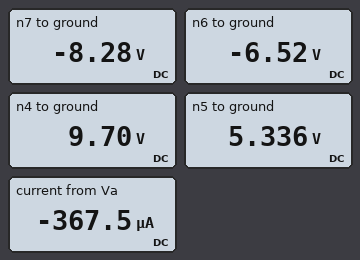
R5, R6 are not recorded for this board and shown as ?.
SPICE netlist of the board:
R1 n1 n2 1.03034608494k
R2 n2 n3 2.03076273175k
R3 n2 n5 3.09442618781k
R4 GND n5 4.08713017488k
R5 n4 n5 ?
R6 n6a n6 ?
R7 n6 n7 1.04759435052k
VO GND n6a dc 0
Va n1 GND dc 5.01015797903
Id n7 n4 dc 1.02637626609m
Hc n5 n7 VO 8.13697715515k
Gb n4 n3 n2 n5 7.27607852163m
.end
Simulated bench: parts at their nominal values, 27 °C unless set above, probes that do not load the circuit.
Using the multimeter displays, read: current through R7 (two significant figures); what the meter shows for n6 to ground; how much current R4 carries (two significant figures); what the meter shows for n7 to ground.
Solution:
1.7 mA
-6.52 V
1.3 mA
-8.28 V
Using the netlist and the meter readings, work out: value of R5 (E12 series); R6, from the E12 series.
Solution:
6.8 kΩ
3.9 kΩ
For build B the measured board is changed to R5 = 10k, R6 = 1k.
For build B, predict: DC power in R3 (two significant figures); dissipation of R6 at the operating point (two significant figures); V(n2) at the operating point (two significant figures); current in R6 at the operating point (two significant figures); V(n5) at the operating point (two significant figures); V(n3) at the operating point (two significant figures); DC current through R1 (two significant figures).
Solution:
950 nW
590 µW
4.6 V
770 µA
4.7 V
3.8 V
380 µA
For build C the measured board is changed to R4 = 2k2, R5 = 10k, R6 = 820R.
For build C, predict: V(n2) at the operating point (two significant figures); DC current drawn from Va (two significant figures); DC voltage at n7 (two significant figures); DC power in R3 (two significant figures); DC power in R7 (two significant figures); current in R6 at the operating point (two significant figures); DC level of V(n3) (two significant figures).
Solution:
3.8 V
1.2 mA
-1.2 V
9.2 µW
420 µW
630 µA
1.3 V
